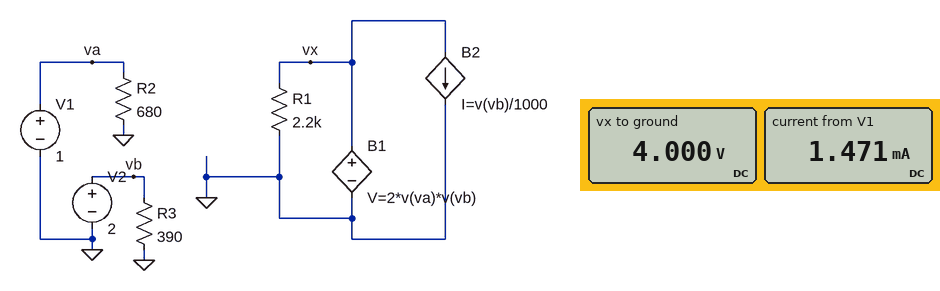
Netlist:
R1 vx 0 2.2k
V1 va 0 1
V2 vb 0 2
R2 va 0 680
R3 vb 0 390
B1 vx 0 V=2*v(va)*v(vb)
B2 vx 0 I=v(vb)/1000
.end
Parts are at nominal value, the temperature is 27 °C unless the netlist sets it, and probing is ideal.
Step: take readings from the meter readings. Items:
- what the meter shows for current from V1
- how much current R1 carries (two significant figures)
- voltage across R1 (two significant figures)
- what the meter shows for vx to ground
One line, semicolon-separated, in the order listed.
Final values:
1.471 mA; 1.8 mA; 4.0 V; 4.000 V
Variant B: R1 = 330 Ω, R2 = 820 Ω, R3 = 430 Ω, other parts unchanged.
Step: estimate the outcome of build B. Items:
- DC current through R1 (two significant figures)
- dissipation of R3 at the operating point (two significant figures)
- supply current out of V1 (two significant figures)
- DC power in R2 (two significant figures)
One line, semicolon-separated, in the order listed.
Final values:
12 mA; 9.3 mW; 1.2 mA; 1.2 mW
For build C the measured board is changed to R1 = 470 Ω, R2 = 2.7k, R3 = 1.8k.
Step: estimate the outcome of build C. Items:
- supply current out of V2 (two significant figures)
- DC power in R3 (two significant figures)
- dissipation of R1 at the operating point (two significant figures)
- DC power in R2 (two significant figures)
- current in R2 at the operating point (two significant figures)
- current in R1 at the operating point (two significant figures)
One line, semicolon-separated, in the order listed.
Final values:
1.1 mA; 2.2 mW; 34 mW; 370 µW; 370 µA; 8.5 mA
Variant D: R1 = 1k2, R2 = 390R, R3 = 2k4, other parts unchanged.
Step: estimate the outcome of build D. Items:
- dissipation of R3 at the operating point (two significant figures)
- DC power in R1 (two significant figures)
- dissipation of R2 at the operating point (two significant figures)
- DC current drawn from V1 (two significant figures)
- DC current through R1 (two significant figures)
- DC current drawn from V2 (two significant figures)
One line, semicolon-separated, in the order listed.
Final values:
1.7 mW; 13 mW; 2.6 mW; 2.6 mA; 3.3 mA; 830 µA
